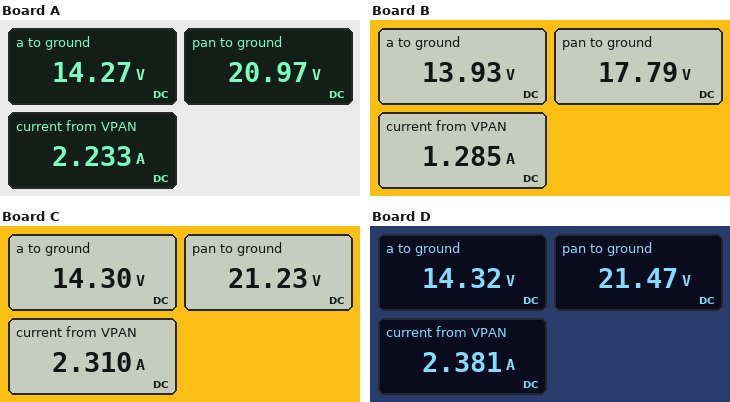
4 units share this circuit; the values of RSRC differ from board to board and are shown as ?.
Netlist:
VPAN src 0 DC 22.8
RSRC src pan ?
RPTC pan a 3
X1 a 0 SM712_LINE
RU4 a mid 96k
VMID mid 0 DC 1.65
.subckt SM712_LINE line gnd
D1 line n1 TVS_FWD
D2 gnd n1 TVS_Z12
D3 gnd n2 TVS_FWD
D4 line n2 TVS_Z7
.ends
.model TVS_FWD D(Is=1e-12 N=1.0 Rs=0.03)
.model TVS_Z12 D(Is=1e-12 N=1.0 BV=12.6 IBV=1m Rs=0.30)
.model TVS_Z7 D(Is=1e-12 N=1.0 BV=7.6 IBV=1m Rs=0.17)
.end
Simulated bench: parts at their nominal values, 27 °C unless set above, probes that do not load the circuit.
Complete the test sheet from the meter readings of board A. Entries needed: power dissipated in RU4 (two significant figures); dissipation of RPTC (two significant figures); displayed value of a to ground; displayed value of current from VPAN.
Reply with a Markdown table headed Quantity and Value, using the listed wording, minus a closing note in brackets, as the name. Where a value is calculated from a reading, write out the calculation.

| Quantity | Value |
|---|---|
| power dissipated in RU4 | (14.27 V - 1.65 V)^2 / 96 kΩ = 1.7 mW |
| dissipation of RPTC | (20.97 V - 14.27 V)^2 / 3 Ω = 15 W |
| displayed value of a to ground | 14.27 V |
| displayed value of current from VPAN | 2.233 A |
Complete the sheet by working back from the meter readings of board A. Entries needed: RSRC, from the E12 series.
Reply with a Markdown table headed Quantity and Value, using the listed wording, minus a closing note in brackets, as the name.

| Quantity | Value |
|---|---|
| RSRC, from the E12 series | 0.82 Ω |
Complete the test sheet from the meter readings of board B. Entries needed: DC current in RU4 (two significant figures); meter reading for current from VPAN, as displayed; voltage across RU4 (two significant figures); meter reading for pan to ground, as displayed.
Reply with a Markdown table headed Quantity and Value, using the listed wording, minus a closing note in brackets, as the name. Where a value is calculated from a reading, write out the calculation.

| Quantity | Value |
|---|---|
| DC current in RU4 | (13.93 V - 1.65 V) / 96 kΩ = 130 µA |
| meter reading for current from VPAN, as displayed | 1.285 A |
| voltage across RU4 | 13.93 V - 1.65 V = 12 V |
| meter reading for pan to ground, as displayed | 17.79 V |
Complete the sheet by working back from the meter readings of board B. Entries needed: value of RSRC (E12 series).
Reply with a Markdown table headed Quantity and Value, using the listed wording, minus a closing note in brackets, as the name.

| Quantity | Value |
|---|---|
| value of RSRC | 3.9 Ω |
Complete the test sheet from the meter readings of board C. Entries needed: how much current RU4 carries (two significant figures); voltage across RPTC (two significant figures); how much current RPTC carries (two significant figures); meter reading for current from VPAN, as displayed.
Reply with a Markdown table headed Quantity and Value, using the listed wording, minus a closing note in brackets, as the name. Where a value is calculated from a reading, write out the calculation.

| Quantity | Value |
|---|---|
| how much current RU4 carries | (14.3 V - 1.65 V) / 96 kΩ = 130 µA |
| voltage across RPTC | 21.23 V - 14.3 V = 6.9 V |
| how much current RPTC carries | (21.23 V - 14.3 V) / 3 Ω = 2.3 A |
| meter reading for current from VPAN, as displayed | 2.310 A |
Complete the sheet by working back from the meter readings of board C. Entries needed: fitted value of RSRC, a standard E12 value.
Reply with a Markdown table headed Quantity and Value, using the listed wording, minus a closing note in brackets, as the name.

| Quantity | Value |
|---|---|
| fitted value of RSRC, a standard E12 value | 0.68 Ω |
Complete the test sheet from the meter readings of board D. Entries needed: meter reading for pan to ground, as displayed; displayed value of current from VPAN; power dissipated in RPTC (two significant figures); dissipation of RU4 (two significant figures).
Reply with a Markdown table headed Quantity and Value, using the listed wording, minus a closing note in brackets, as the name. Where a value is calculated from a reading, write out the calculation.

| Quantity | Value |
|---|---|
| meter reading for pan to ground, as displayed | 21.47 V |
| displayed value of current from VPAN | 2.381 A |
| power dissipated in RPTC | (21.47 V - 14.32 V)^2 / 3 Ω = 17 W |
| dissipation of RU4 | (14.32 V - 1.65 V)^2 / 96 kΩ = 1.7 mW |
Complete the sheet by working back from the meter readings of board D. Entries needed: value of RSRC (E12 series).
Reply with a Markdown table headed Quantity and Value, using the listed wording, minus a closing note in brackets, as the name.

| Quantity | Value |
|---|---|
| value of RSRC | 0.56 Ω |
